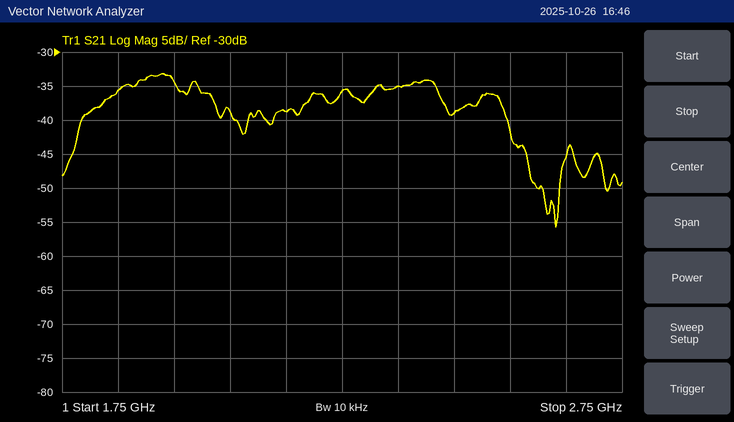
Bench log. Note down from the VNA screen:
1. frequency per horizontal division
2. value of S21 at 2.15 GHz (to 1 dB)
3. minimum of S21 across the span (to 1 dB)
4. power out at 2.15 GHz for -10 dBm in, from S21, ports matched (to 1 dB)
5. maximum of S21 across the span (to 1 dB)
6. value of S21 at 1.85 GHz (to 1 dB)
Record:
100 MHz
-39 dB
-56 dB
-49 dBm
-33 dB
-36 dB
